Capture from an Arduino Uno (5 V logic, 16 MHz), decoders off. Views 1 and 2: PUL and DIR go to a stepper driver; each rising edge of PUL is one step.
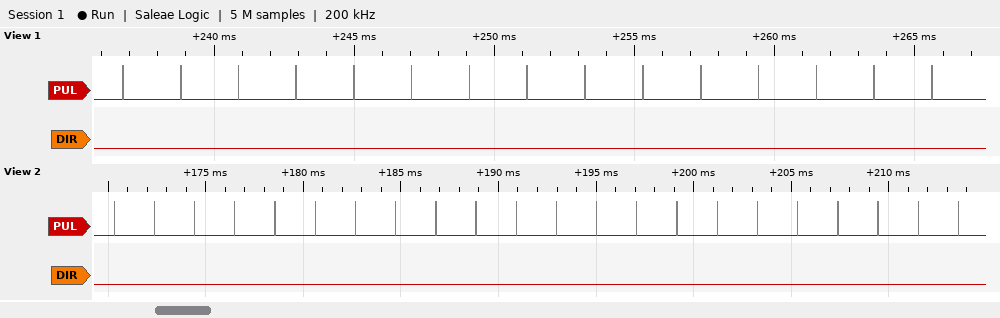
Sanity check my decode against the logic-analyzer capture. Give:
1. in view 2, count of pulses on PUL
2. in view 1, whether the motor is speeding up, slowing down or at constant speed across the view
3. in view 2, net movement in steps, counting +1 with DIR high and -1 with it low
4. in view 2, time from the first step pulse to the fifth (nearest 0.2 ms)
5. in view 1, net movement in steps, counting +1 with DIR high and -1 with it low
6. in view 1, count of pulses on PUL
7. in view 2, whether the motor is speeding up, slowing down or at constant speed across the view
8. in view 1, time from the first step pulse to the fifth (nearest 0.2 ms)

22
constant speed
-22
8.2 ms
-15
15
constant speed
8.2 ms
